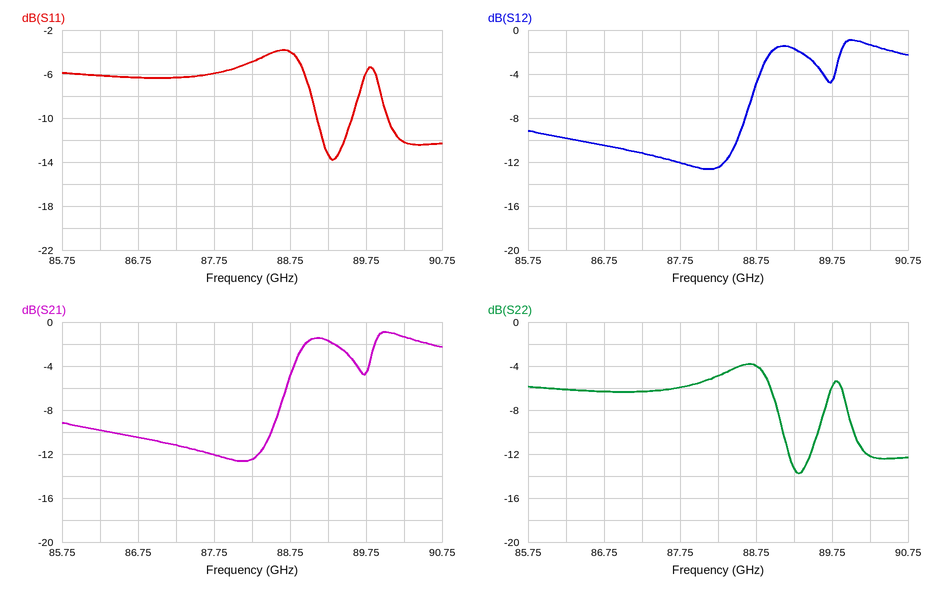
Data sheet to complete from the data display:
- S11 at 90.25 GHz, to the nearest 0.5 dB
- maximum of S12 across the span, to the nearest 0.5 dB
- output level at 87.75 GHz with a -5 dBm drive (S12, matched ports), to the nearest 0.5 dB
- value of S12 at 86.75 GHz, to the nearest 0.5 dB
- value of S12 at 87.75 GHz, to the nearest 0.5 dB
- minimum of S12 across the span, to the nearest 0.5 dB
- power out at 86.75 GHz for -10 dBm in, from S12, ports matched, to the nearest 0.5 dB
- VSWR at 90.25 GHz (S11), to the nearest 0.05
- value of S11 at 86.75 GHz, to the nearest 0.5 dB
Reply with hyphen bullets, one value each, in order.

- -12.0 dB
- -1.0 dB
- -17.0 dBm
- -10.5 dB
- -12.0 dB
- -12.5 dB
- -20.5 dBm
- 1.65
- -6.5 dB
